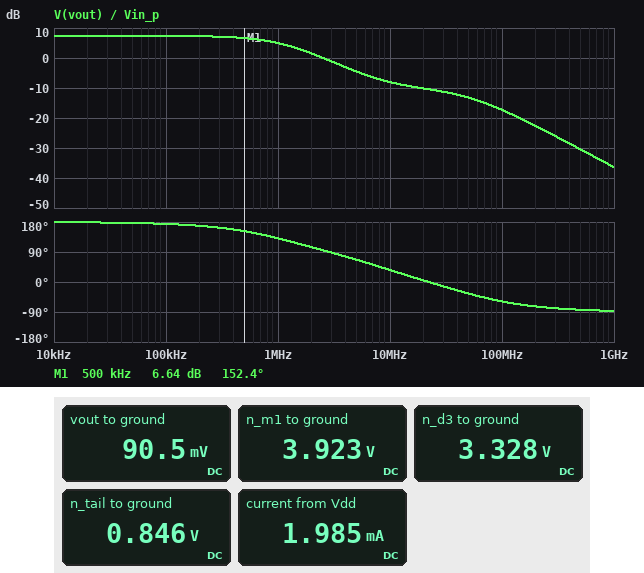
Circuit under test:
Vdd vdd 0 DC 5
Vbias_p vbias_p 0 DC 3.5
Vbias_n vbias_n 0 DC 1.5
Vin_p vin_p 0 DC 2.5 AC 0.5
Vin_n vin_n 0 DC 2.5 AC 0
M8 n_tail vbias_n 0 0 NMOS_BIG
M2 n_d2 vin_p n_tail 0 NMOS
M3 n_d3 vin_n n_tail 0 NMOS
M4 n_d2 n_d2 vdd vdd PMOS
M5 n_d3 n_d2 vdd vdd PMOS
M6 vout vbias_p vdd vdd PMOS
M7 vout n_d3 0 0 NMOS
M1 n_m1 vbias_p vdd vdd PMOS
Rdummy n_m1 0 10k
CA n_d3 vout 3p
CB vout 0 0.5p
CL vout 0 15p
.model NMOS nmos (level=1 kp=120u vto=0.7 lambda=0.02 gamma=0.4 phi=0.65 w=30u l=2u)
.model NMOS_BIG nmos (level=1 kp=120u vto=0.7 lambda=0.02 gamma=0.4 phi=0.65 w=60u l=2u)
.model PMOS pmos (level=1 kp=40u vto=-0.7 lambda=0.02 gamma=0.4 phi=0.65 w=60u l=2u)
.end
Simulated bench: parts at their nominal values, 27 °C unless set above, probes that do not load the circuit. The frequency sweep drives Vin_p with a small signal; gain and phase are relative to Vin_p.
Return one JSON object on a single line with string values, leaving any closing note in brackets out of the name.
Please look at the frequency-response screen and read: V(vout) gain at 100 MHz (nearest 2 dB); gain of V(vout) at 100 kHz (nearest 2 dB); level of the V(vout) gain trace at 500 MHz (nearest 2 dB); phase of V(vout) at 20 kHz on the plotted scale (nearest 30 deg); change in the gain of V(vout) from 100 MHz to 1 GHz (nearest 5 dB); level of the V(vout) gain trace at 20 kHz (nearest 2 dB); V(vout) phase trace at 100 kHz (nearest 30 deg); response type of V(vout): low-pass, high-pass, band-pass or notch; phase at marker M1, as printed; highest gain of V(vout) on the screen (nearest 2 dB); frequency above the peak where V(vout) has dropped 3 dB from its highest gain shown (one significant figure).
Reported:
{"V(vout) gain at 100 MHz": "-18 dB", "gain of V(vout) at 100 kHz": "8 dB", "level of the V(vout) gain trace at 500 MHz": "-30 dB", "phase of V(vout) at 20 kHz on the plotted scale": "180 deg", "change in the gain of V(vout) from 100 MHz to 1 GHz": "-20 dB", "level of the V(vout) gain trace at 20 kHz": "8 dB", "V(vout) phase trace at 100 kHz": "180 deg", "response type of V(vout): low-pass, high-pass, band-pass or notch": "low-pass", "phase at marker M1, as printed": "152.4 deg", "highest gain of V(vout) on the screen": "8 dB", "frequency above the peak where V(vout) has dropped 3 dB from its highest gain shown": "1 MHz"}
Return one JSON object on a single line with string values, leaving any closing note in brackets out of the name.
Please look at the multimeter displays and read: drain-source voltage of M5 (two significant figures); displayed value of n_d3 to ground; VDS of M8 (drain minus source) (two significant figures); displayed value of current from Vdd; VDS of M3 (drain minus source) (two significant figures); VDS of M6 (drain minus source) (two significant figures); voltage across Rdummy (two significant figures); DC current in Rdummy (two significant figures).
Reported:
{"drain-source voltage of M5": "-1.7 V", "displayed value of n_d3 to ground": "3.328 V", "VDS of M8 (drain minus source)": "850 mV", "displayed value of current from Vdd": "1.985 mA", "VDS of M3 (drain minus source)": "2.5 V", "VDS of M6 (drain minus source)": "-4.9 V", "voltage across Rdummy": "3.9 V", "DC current in Rdummy": "390 µA"}
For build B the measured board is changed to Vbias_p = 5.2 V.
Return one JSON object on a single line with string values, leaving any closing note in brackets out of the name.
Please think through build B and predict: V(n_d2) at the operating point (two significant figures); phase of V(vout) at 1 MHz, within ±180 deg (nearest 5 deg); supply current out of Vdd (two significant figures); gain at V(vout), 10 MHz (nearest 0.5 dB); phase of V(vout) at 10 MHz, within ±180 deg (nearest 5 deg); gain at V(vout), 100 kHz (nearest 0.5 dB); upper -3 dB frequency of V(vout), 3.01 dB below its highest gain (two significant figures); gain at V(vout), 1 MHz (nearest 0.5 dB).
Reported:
{"V(n_d2) at the operating point": "3.3 V", "phase of V(vout) at 1 MHz, within ±180 deg": "50 deg", "supply current out of Vdd": "1.2 mA", "gain at V(vout), 10 MHz": "-10.5 dB", "phase of V(vout) at 10 MHz, within ±180 deg": "-5 deg", "gain at V(vout), 100 kHz": "-31.5 dB", "upper -3 dB frequency of V(vout), 3.01 dB below its highest gain": "51 MHz", "gain at V(vout), 1 MHz": "-14.0 dB"}
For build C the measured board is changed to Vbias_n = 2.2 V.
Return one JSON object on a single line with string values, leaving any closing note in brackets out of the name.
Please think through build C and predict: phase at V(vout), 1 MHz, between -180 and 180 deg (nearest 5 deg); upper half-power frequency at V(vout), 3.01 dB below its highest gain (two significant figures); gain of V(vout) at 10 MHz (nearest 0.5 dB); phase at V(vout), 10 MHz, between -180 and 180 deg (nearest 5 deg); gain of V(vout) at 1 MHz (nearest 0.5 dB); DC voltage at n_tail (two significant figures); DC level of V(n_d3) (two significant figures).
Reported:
{"phase at V(vout), 1 MHz, between -180 and 180 deg": "150 deg", "upper half-power frequency at V(vout), 3.01 dB below its highest gain": "2.4 MHz", "gain of V(vout) at 10 MHz": "-3.0 dB", "phase at V(vout), 10 MHz, between -180 and 180 deg": "45 deg", "gain of V(vout) at 1 MHz": "6.5 dB", "DC voltage at n_tail": "550 mV", "DC level of V(n_d3)": "2.9 V"}
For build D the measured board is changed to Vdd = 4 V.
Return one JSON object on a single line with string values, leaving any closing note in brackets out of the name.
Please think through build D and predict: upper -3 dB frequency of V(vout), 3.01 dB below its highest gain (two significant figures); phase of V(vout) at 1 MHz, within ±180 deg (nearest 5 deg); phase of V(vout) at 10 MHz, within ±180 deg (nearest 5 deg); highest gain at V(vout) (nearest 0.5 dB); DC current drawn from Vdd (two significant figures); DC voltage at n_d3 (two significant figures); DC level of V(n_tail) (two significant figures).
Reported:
{"upper -3 dB frequency of V(vout), 3.01 dB below its highest gain": "33 MHz", "phase of V(vout) at 1 MHz, within ±180 deg": "50 deg", "phase of V(vout) at 10 MHz, within ±180 deg": "-10 deg", "highest gain at V(vout)": "-6.5 dB", "DC current drawn from Vdd": "1.2 mA", "DC voltage at n_d3": "2.3 V", "DC level of V(n_tail)": "840 mV"}
